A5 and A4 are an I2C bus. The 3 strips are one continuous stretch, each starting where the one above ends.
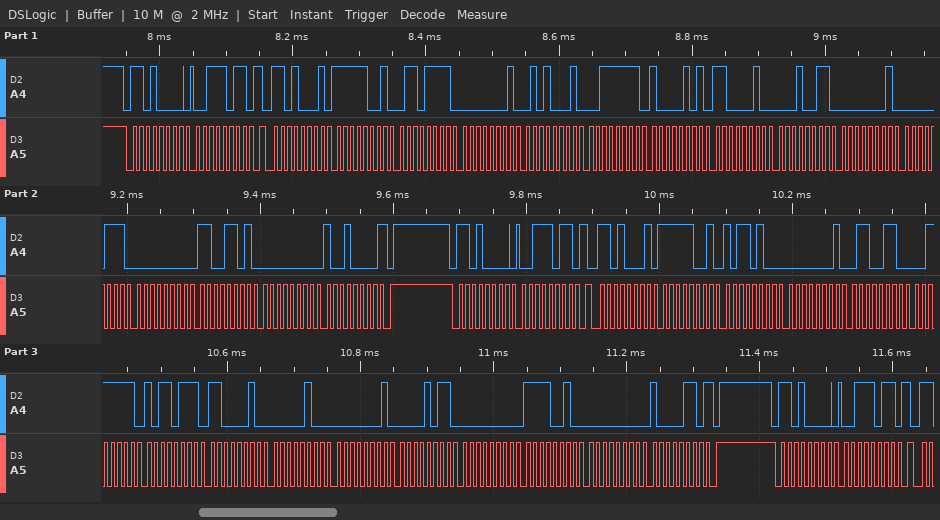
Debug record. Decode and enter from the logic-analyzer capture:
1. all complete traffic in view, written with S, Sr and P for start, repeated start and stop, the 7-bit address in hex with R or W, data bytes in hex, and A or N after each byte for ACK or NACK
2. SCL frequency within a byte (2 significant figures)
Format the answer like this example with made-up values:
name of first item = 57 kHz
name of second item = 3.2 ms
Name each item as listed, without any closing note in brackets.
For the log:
all complete traffic in view, written with S, Sr and P for start, repeated start and stop, the 7-bit address in hex with R or W, data bytes in hex, and A or N after each byte for ACK or NACK = S 68W A 3B A Sr 68R A F9 A 6F A 01 A 51 A 3F A 85 A C2 A 13 A 01 A 07 A 00 A CD A 00 A 90 N P S 68W A 3B A Sr 68R A F9 A B4 A 01 A 66 A 3F A B7 A C2 A 04 A 01 A 0B A 00 A F2 A 00 A 86 N P S 68W A 3B A
SCL frequency within a byte = 100 kHz
